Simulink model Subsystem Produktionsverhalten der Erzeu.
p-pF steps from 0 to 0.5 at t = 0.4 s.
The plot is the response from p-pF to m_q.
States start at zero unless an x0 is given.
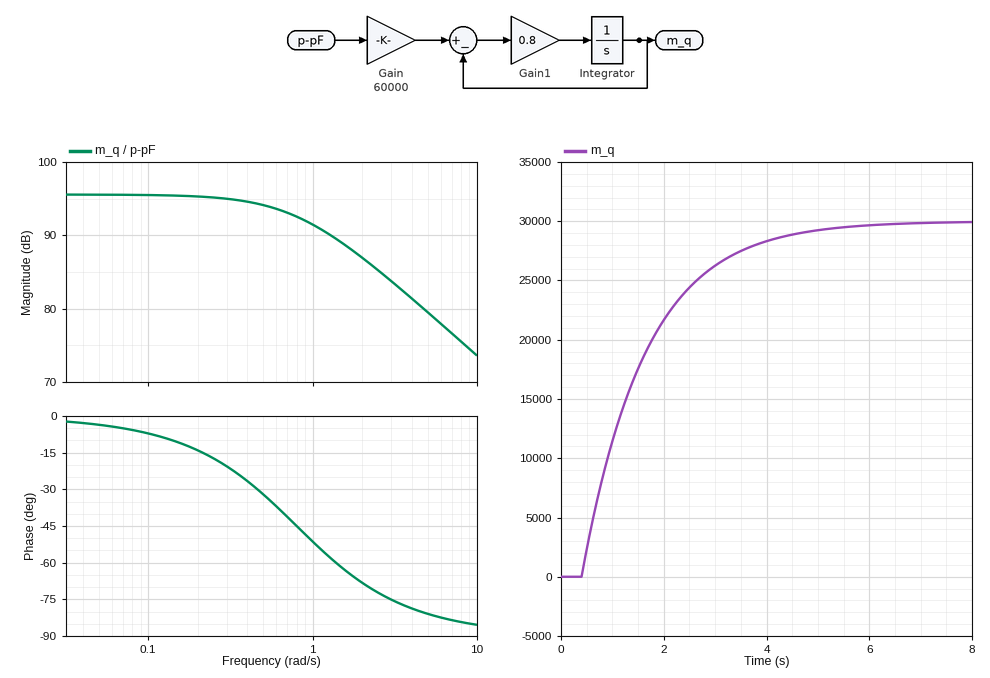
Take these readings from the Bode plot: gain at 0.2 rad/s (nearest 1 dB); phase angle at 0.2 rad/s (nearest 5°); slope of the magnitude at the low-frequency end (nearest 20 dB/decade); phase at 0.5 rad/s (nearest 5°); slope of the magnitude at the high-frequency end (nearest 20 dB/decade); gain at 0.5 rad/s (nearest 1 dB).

95 dB
-15°
0 dB/decade
-30°
-20 dB/decade
94 dB
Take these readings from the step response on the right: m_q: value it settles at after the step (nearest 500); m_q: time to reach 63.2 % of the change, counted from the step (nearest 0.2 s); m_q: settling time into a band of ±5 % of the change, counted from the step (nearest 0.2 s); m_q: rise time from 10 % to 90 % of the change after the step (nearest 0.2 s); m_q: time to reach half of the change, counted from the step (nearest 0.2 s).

30000
1.2 s
3.8 s
2.8 s
0.8 s
